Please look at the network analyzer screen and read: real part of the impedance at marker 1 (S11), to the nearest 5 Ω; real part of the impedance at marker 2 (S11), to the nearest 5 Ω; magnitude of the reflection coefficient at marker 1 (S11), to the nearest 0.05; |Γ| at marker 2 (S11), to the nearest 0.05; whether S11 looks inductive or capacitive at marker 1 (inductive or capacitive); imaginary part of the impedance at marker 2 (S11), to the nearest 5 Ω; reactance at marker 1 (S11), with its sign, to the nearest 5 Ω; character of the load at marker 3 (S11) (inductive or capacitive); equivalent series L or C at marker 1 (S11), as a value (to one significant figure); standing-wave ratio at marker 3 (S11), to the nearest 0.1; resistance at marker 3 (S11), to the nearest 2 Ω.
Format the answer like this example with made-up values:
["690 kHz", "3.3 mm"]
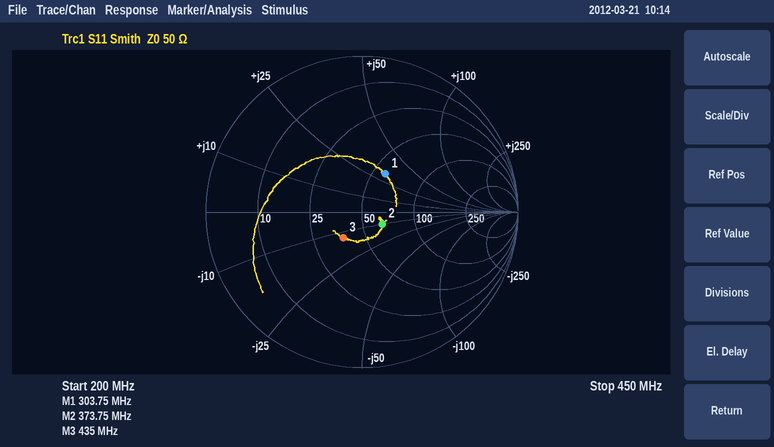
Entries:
["60 Ω", "65 Ω", "0.30", "0.15", "inductive", "-10 Ω", "+30 Ω", "capacitive", "20 nH", "1.5", "38 Ω"]
